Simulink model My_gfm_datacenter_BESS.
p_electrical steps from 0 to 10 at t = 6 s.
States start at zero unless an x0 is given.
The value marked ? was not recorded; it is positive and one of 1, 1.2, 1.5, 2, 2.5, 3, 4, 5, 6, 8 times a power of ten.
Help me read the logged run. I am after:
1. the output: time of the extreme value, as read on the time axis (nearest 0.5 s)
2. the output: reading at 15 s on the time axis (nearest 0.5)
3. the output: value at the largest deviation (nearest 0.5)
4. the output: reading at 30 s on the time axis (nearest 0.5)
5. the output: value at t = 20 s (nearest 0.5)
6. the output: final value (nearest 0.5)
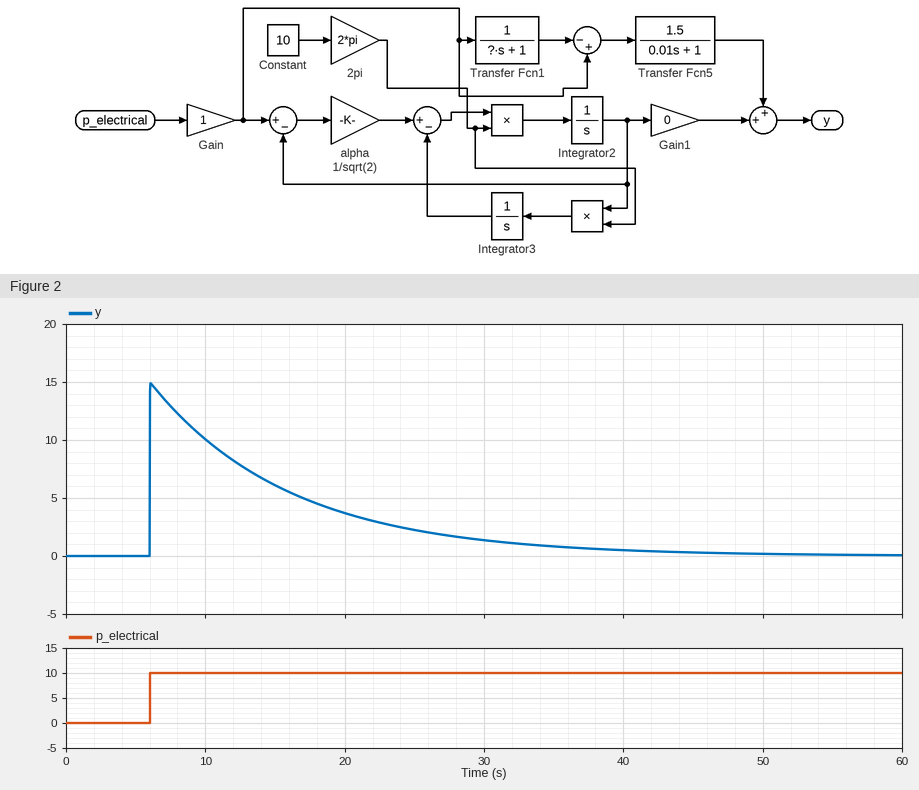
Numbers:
6.0 s
6.0
15.0
1.5
3.5
0.0
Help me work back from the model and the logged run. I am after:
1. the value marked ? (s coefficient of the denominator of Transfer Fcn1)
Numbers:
10
